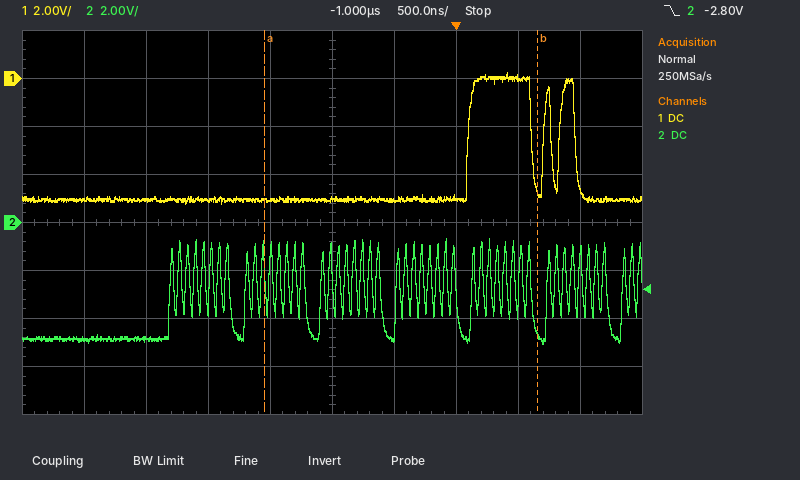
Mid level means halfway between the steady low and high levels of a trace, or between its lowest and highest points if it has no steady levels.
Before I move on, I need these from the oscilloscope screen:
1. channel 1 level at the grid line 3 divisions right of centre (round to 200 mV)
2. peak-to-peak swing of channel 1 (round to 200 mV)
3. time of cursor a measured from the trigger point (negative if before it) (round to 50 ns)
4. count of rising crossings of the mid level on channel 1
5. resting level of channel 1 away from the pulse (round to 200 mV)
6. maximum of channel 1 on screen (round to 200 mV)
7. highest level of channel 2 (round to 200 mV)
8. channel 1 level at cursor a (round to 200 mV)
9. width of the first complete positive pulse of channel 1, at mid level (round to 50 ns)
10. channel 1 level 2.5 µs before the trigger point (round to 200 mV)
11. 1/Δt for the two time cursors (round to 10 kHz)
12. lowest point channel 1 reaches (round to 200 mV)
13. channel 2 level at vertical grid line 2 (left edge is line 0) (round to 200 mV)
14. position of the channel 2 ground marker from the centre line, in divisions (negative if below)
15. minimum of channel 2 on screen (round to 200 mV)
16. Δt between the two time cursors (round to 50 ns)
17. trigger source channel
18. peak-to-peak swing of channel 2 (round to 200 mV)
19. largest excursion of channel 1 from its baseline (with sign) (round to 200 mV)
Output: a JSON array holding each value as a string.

["0.0 V", "5.4 V", "-1.55 µs", "3", "-5.0 V", "200 mV", "-600 mV", "-5.0 V", "500 ns", "-5.0 V", "450 kHz", "-5.2 V", "-4.8 V", "0.0 div", "-5.0 V", "2.20 µs", "channel 2", "4.4 V", "+5.2 V"]
